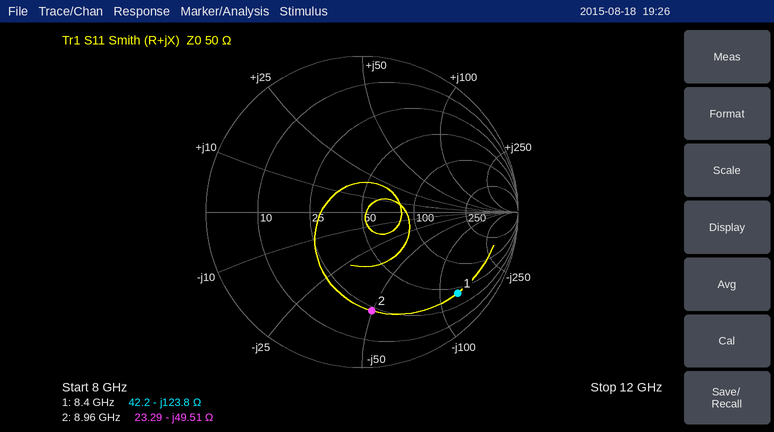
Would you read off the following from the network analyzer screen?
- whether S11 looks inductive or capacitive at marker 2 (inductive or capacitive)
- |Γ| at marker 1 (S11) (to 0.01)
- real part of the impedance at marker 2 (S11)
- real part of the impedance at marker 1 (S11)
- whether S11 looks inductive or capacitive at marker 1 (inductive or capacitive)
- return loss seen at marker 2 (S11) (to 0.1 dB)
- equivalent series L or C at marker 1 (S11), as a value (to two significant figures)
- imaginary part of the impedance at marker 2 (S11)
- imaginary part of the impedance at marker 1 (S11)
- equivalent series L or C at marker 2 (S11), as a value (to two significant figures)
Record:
capacitive
0.80
23.29 Ω
42.2 Ω
capacitive
3.9 dB
150 fF
-49.51 Ω
-123.8 Ω
360 fF
